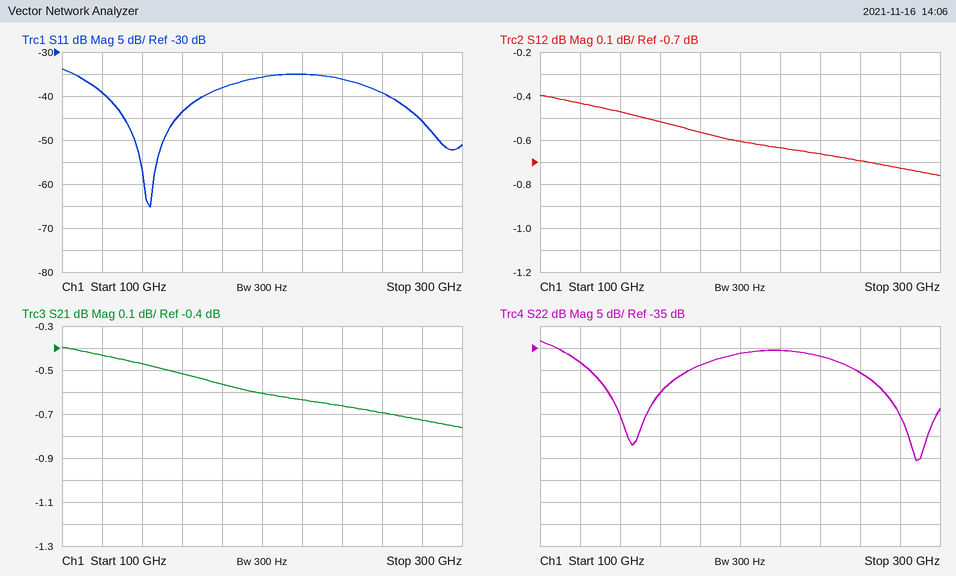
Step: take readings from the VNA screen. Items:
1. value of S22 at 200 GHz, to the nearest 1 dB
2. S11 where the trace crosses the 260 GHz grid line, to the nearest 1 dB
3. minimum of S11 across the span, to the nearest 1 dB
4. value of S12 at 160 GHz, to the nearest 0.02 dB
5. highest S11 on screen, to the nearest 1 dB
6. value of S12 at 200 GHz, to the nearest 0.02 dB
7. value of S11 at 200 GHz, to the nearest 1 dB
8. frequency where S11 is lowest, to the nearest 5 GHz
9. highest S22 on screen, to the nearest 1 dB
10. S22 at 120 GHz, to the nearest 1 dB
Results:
-36 dB
-39 dB
-65 dB
-0.52 dB
-34 dB
-0.60 dB
-36 dB
145 GHz
-33 dB
-38 dB
